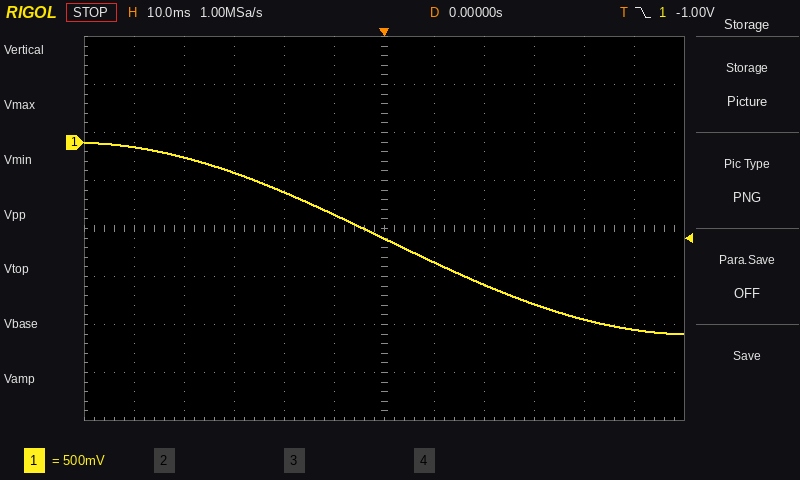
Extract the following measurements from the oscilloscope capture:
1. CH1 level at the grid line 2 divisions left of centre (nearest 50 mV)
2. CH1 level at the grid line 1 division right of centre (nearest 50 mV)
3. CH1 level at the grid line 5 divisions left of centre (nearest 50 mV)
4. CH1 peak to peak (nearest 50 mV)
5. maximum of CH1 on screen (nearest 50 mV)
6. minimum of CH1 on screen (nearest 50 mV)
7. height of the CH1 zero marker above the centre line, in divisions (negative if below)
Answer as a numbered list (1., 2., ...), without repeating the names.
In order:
1. -500 mV
2. -1.25 V
3. -50 mV
4. 2.00 V
5. 0 mV
6. -2.00 V
7. +1.8 div
